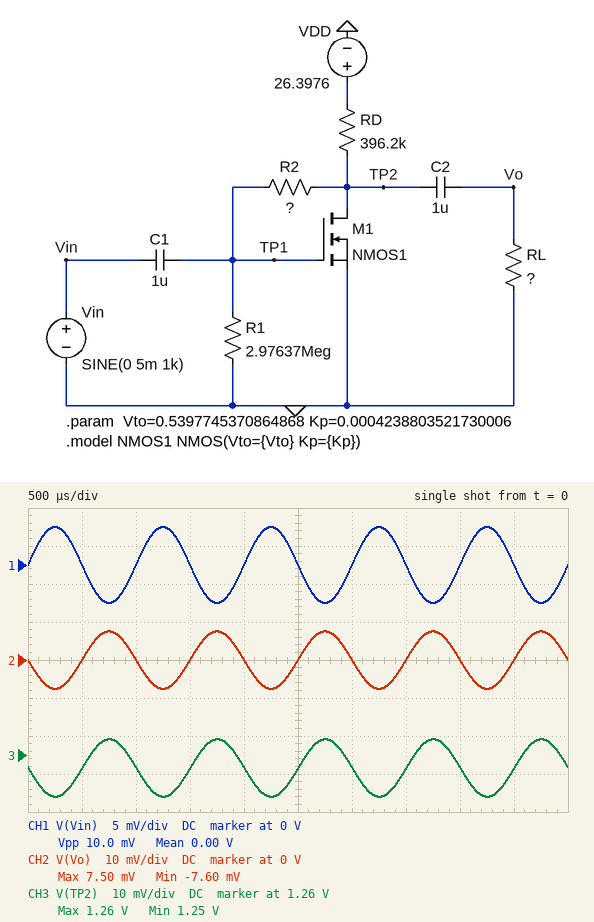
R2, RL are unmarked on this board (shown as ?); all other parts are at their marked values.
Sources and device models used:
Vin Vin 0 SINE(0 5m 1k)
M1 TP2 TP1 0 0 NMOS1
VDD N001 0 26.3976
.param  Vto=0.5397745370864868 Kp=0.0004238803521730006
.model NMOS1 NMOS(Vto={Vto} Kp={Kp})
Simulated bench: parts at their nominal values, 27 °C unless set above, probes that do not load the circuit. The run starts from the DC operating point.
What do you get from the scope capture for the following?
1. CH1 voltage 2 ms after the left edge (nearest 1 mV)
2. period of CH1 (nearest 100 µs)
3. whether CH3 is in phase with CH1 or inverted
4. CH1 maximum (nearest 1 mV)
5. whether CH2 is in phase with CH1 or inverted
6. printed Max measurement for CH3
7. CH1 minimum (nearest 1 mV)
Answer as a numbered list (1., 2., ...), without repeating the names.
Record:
1. 0 V
2. 1.0 ms
3. inverted
4. 5 mV
5. inverted
6. 1.26 V
7. -5 mV
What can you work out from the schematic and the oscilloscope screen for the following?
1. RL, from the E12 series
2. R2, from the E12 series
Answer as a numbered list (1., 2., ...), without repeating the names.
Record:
1. 6.8 kΩ
2. 470 kΩ
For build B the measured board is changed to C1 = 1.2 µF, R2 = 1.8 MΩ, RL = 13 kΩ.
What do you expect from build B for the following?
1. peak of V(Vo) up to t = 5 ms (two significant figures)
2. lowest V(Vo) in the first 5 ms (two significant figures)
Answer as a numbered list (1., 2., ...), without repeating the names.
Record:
1. 14 mV
2. -14 mV
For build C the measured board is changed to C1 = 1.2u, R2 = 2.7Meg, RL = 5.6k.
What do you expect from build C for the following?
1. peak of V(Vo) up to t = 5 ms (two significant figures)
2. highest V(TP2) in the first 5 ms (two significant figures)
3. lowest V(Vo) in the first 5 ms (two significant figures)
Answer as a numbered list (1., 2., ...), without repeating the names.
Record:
1. 6.2 mV
2. 2.1 V
3. -6.3 mV
